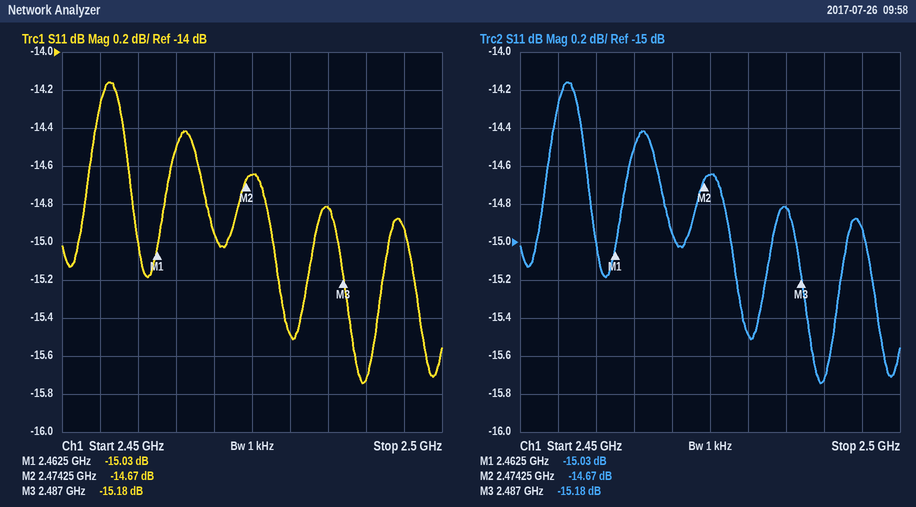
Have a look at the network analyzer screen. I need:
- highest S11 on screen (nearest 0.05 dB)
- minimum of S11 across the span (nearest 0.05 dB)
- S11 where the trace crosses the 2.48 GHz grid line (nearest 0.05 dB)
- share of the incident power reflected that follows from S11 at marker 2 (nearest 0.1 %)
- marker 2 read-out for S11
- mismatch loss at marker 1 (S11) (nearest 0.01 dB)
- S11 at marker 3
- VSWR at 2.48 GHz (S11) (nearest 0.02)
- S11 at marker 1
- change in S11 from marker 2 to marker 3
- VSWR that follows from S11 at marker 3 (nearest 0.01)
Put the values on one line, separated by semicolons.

-14.15 dB; -15.75 dB; -15.50 dB; 3.4 %; -14.67 dB; 0.14 dB; -15.18 dB; 1.40; -15.03 dB; -0.51 dB; 1.42
